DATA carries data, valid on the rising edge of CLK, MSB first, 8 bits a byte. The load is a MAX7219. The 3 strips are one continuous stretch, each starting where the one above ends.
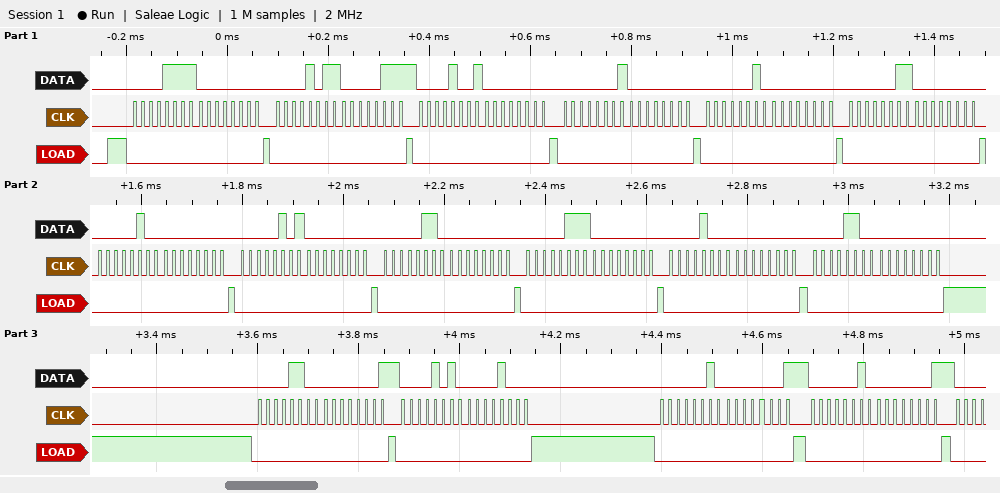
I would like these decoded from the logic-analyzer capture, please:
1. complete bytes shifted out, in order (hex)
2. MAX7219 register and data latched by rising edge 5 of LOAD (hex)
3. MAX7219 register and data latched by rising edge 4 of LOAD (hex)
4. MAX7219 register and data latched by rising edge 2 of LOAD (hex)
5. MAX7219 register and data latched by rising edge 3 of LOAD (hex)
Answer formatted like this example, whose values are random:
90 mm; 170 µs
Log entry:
0F 00 0B 07 09 00 01 00 02 00 03 00 04 00 05 00 06 00 07 00 08 00 0C 00 0C 01 0A 08 02 01 02 01; register 0x1, data 0x00; register 0x9, data 0x00; register 0xF, data 0x00; register 0xB, data 0x07
